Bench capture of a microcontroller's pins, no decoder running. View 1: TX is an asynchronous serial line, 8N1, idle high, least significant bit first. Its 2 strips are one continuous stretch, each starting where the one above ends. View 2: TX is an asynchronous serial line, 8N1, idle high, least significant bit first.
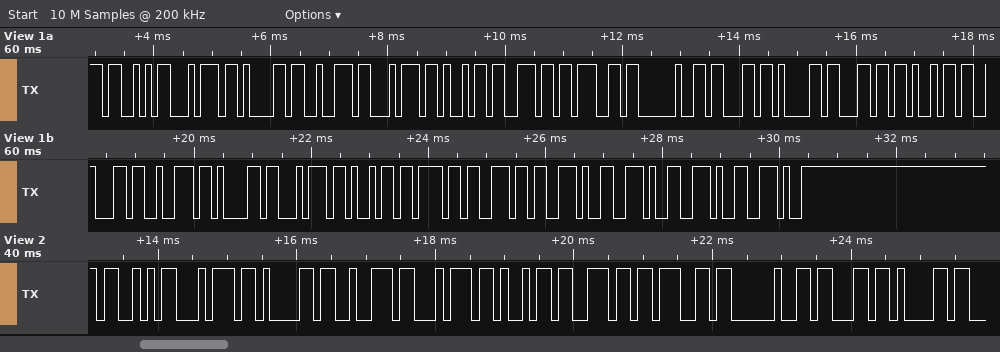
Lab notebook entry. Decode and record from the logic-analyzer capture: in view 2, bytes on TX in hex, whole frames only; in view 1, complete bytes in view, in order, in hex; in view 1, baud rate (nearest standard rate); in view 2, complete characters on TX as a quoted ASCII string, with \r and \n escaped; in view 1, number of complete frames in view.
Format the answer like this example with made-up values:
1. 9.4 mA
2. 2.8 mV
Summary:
1. 0x53 0x74 0x61 0x72 0x74 0x69 0x6E 0x67 0x20 0x63 0x61
2. 53 74 61 72 74 69 6E 67 20 63 61 6C 69 62 72 61 74 69 6F 6E 2E 2E 2E 2E
3. 9600 baud
4. "Starting ca"
5. 24
